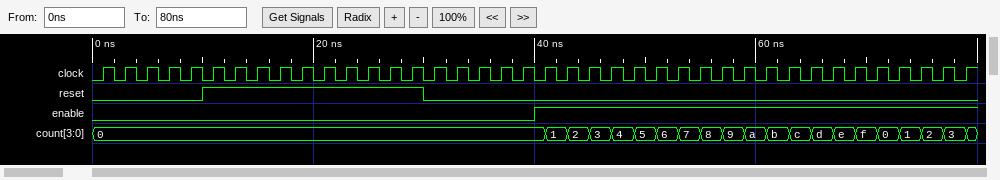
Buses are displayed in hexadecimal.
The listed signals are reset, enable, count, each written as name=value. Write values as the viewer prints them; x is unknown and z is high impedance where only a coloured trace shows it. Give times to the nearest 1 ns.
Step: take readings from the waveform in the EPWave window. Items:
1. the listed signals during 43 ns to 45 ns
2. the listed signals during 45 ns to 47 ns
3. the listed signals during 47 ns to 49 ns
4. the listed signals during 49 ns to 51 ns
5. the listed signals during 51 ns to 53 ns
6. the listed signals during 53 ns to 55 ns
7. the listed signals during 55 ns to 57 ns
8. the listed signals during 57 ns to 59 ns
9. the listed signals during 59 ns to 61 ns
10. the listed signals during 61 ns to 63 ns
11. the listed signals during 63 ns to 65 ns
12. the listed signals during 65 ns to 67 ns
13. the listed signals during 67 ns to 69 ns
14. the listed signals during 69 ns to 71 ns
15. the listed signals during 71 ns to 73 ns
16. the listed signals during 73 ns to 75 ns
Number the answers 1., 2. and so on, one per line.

1. reset=0, enable=1, count=2
2. reset=0, enable=1, count=3
3. reset=0, enable=1, count=4
4. reset=0, enable=1, count=5
5. reset=0, enable=1, count=6
6. reset=0, enable=1, count=7
7. reset=0, enable=1, count=8
8. reset=0, enable=1, count=9
9. reset=0, enable=1, count=a
10. reset=0, enable=1, count=b
11. reset=0, enable=1, count=c
12. reset=0, enable=1, count=d
13. reset=0, enable=1, count=e
14. reset=0, enable=1, count=f
15. reset=0, enable=1, count=0
16. reset=0, enable=1, count=1
